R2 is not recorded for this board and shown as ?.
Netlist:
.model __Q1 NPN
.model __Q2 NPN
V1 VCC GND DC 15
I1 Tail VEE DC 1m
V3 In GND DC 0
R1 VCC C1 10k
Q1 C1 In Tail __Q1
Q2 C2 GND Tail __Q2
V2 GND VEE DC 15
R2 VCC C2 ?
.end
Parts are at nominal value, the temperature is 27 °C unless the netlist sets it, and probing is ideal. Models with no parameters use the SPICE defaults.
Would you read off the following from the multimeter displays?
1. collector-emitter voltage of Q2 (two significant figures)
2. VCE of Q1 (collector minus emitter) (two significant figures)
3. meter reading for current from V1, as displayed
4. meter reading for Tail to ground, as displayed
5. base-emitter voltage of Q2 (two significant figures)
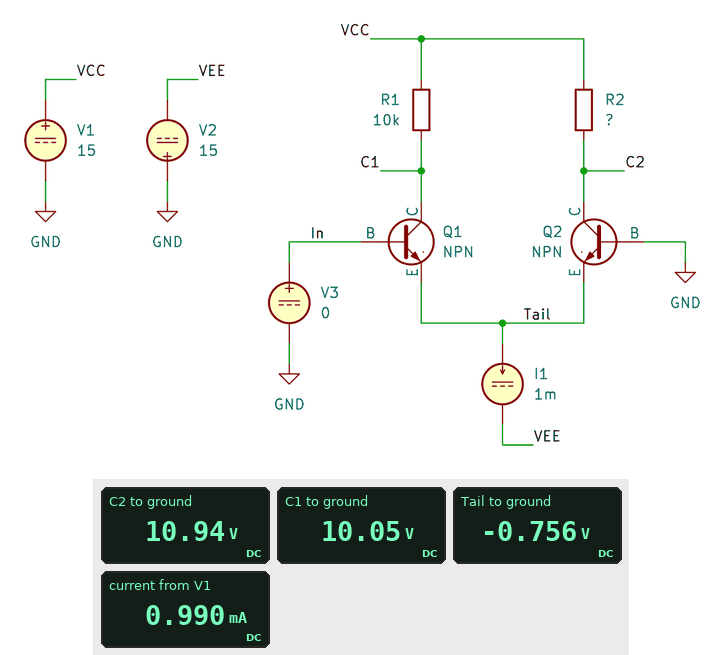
12 V
11 V
0.990 mA
-0.756 V
760 mV
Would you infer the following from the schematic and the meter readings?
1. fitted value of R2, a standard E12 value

8.2 kΩ
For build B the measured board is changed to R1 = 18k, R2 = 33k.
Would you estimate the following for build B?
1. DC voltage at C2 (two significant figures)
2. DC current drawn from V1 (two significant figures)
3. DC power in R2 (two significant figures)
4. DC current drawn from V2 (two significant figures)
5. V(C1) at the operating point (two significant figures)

-660 mV
980 µA
7.4 mW
1.0 mA
6.0 V
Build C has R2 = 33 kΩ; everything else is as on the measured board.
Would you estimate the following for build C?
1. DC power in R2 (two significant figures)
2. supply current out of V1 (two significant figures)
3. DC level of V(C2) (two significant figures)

7.4 mW
980 µA
-660 mV
